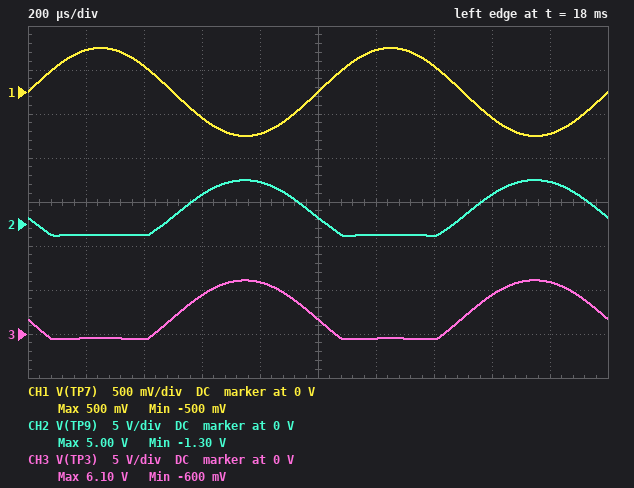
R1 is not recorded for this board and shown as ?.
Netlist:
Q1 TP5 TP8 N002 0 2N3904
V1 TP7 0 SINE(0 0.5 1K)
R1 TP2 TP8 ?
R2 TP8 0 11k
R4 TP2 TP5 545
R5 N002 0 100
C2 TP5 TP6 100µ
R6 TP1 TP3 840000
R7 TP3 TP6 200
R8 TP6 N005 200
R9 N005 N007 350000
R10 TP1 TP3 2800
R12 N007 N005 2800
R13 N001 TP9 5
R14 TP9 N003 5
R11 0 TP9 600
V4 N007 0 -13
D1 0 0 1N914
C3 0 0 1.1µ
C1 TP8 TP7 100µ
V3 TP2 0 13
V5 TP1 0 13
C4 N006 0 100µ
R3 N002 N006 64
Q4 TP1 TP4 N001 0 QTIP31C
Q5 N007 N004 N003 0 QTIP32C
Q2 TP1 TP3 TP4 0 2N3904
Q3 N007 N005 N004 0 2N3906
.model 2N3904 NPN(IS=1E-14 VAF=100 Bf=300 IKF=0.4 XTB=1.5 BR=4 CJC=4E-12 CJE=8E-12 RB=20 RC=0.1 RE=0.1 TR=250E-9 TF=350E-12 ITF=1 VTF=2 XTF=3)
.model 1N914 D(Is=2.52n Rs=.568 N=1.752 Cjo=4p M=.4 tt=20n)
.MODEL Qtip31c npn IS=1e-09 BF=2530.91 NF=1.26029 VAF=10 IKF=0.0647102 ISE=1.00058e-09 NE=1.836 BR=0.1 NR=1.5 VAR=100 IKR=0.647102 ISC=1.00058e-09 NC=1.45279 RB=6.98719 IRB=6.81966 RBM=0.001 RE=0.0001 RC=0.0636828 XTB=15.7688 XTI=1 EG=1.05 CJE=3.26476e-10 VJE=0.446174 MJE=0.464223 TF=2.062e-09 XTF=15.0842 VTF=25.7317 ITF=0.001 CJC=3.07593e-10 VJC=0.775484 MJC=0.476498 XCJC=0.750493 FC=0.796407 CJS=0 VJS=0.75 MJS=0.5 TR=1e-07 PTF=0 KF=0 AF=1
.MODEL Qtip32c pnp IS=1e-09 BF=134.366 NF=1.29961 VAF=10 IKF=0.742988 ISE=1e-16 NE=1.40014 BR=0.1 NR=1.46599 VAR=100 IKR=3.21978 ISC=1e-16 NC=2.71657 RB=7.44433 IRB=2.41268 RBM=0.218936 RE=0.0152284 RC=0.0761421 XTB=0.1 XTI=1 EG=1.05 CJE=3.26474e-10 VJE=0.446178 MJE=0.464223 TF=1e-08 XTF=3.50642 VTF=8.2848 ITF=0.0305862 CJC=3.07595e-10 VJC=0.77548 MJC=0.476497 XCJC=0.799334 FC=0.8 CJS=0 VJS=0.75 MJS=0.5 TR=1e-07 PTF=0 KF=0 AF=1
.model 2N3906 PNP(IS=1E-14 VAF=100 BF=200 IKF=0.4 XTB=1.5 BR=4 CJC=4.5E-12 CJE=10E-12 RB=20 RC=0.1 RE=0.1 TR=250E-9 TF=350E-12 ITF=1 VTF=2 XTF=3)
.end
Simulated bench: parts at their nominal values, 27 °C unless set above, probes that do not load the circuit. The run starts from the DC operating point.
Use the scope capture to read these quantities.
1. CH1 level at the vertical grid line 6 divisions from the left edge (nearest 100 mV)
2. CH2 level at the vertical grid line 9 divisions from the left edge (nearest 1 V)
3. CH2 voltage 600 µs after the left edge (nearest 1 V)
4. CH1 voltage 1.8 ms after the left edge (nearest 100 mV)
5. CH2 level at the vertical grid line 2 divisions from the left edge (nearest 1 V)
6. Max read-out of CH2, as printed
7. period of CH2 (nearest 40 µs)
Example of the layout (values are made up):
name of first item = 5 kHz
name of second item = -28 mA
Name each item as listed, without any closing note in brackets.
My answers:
CH1 level at the vertical grid line 6 divisions from the left edge = 500 mV
CH2 level at the vertical grid line 9 divisions from the left edge = 5 V
CH2 voltage 600 µs after the left edge = 3 V
CH1 voltage 1.8 ms after the left edge = -500 mV
CH2 level at the vertical grid line 2 divisions from the left edge = -1 V
Max read-out of CH2, as printed = 5.00 V
period of CH2 = 1.00 ms
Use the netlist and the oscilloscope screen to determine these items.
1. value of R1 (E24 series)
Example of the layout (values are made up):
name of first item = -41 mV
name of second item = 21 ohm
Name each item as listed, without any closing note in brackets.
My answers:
value of R1 = 36 kΩ
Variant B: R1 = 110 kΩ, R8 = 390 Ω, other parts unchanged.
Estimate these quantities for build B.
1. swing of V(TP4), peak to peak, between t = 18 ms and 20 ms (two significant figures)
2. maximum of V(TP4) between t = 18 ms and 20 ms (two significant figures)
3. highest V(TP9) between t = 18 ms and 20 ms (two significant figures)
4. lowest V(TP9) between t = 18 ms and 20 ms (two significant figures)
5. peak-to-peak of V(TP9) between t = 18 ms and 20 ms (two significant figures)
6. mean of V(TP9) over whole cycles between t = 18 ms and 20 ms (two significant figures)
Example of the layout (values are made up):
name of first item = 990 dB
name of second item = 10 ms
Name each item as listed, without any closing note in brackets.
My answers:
swing of V(TP4), peak to peak, between t = 18 ms and 20 ms = 5.2 V
maximum of V(TP4) between t = 18 ms and 20 ms = 2.1 V
highest V(TP9) between t = 18 ms and 20 ms = 1.4 V
lowest V(TP9) between t = 18 ms and 20 ms = -3.7 V
peak-to-peak of V(TP9) between t = 18 ms and 20 ms = 5.1 V
mean of V(TP9) over whole cycles between t = 18 ms and 20 ms = -410 mV
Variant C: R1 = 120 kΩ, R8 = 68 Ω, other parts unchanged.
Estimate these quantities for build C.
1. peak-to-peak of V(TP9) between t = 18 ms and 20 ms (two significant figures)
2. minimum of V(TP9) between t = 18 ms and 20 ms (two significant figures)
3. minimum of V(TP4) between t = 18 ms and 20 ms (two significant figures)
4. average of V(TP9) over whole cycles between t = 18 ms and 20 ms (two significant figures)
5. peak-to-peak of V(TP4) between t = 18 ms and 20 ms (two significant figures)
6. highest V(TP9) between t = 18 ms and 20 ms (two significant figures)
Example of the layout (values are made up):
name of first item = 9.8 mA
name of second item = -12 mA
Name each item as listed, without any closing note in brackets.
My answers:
peak-to-peak of V(TP9) between t = 18 ms and 20 ms = 4.2 V
minimum of V(TP9) between t = 18 ms and 20 ms = -3.4 V
minimum of V(TP4) between t = 18 ms and 20 ms = -3.1 V
average of V(TP9) over whole cycles between t = 18 ms and 20 ms = -540 mV
peak-to-peak of V(TP4) between t = 18 ms and 20 ms = 4.3 V
highest V(TP9) between t = 18 ms and 20 ms = 810 mV
